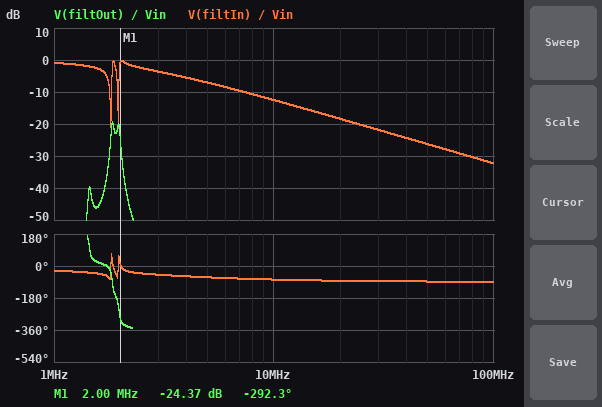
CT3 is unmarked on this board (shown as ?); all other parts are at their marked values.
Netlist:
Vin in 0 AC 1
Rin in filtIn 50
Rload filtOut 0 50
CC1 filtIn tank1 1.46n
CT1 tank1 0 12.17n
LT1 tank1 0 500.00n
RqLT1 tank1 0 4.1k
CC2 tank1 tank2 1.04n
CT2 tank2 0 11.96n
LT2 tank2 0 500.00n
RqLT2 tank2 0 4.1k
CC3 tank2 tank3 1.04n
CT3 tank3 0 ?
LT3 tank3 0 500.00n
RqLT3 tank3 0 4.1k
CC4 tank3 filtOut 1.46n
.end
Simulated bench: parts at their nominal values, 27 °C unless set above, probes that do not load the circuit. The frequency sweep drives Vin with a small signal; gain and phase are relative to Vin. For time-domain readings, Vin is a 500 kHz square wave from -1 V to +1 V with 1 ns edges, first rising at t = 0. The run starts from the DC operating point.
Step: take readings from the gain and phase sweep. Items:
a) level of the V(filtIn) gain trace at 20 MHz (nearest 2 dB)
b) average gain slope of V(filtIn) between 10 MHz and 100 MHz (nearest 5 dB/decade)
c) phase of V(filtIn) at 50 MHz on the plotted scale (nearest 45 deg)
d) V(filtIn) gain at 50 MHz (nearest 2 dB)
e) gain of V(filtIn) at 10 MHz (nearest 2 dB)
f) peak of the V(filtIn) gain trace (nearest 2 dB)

-18 dB
-20 dB/decade
-90 deg
-26 dB
-12 dB
0 dB
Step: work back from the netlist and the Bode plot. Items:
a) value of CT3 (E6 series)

22 nF
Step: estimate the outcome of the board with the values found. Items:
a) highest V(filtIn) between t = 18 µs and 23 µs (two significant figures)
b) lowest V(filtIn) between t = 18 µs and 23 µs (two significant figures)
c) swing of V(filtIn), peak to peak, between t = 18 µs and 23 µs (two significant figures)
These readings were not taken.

1.1 V
-1.1 V
2.1 V
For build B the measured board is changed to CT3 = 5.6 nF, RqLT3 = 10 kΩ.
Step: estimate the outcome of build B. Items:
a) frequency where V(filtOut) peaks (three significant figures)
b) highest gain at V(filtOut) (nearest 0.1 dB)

1.96 MHz
-15.9 dB
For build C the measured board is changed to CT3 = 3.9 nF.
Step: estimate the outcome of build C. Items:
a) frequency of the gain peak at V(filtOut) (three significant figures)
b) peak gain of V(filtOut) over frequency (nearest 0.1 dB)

1.96 MHz
-17.9 dB
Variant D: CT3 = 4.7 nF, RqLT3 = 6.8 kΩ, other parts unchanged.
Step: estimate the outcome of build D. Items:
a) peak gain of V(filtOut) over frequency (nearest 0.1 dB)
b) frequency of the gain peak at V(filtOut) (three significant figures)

-17.0 dB
1.96 MHz
